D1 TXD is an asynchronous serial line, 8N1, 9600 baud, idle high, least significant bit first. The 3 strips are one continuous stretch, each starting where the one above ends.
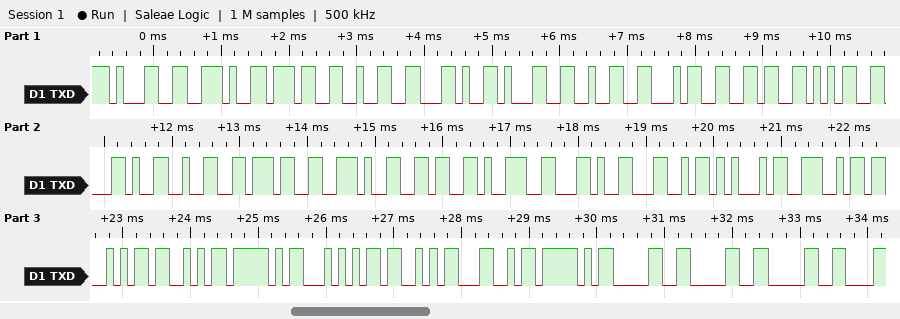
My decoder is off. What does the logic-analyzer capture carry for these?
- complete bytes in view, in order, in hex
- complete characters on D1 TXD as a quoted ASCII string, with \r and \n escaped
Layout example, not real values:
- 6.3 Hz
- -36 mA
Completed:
- 31 2E 37 32 2C 31 32 34 36 35 2C 32 37 2E 36 39 2C 4C 45 4E 53 53 5F 54 53 4C 5F 30 30 30
- "1.72,12465,27.69,LENSS_TSL_000"
